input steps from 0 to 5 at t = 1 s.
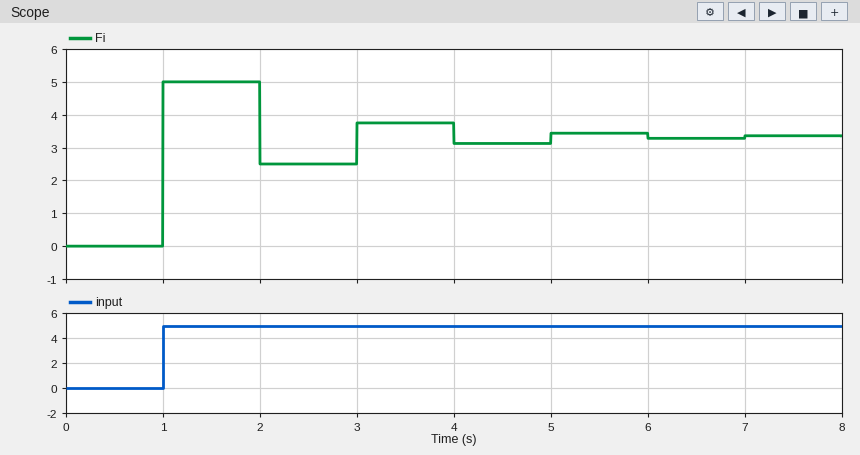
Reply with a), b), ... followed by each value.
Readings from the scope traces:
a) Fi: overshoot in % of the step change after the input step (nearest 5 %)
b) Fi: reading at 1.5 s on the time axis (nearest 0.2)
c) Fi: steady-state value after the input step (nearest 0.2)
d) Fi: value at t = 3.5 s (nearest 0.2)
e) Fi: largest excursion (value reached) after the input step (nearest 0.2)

a) 50 %
b) 5.0
c) 3.4
d) 3.8
e) 5.0
